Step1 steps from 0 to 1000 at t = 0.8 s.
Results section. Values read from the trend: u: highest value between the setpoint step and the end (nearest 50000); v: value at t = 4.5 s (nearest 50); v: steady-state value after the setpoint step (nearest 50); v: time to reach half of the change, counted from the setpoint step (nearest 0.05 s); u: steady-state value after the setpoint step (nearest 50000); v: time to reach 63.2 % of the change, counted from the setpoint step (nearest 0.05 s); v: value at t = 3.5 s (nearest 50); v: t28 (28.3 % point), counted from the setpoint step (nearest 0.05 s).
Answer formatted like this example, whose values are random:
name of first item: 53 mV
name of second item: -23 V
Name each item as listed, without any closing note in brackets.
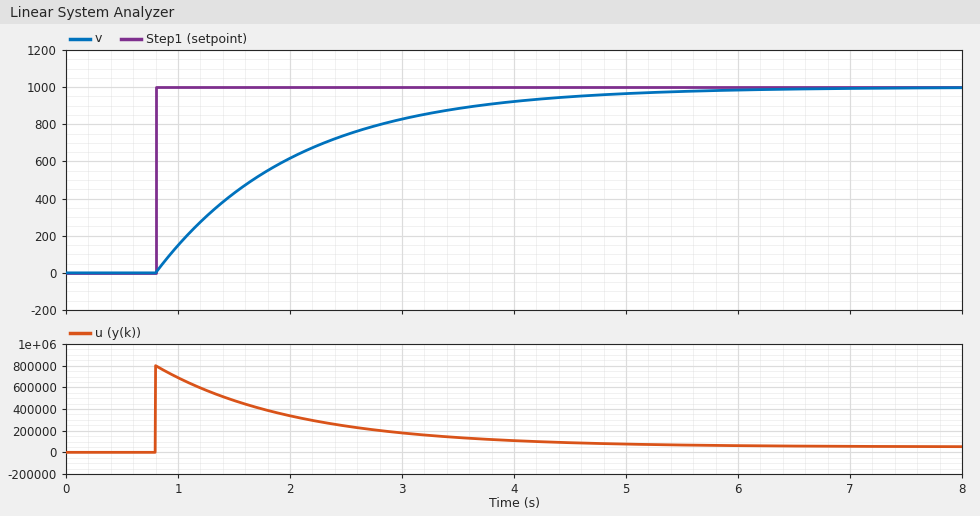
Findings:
u: highest value between the setpoint step and the end: 800000
v: value at t = 4.5 s: 950
v: steady-state value after the setpoint step: 1000
v: time to reach half of the change, counted from the setpoint step: 0.85 s
u: steady-state value after the setpoint step: 50000
v: time to reach 63.2 % of the change, counted from the setpoint step: 1.25 s
v: value at t = 3.5 s: 900
v: t28 (28.3 % point), counted from the setpoint step: 0.40 s
